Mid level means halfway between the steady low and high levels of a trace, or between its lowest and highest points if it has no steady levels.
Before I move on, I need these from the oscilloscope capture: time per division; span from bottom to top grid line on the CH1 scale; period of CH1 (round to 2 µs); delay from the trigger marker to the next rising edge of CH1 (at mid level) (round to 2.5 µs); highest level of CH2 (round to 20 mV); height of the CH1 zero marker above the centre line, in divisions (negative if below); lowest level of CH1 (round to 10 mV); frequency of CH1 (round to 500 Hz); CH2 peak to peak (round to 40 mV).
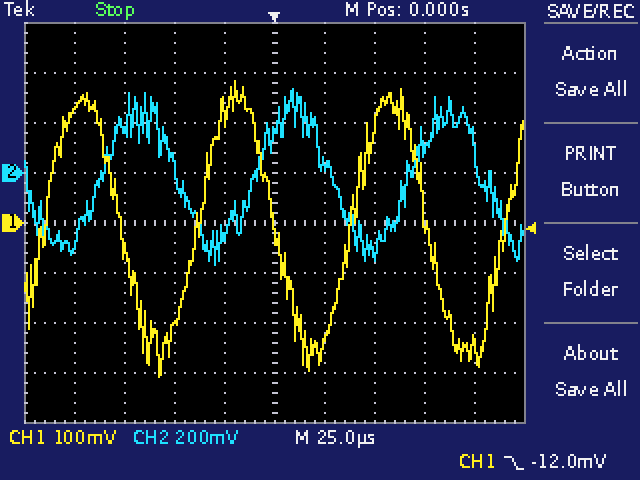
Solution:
25 µs
800 mV
76 µs
37.5 µs
340 mV
0.0 div
-310 mV
13.0 kHz
720 mV
